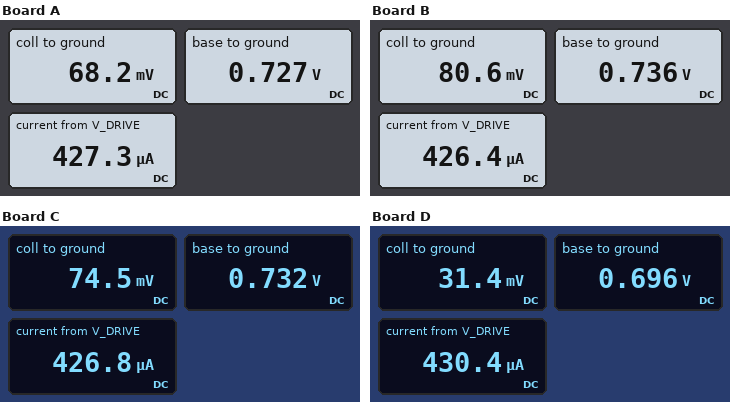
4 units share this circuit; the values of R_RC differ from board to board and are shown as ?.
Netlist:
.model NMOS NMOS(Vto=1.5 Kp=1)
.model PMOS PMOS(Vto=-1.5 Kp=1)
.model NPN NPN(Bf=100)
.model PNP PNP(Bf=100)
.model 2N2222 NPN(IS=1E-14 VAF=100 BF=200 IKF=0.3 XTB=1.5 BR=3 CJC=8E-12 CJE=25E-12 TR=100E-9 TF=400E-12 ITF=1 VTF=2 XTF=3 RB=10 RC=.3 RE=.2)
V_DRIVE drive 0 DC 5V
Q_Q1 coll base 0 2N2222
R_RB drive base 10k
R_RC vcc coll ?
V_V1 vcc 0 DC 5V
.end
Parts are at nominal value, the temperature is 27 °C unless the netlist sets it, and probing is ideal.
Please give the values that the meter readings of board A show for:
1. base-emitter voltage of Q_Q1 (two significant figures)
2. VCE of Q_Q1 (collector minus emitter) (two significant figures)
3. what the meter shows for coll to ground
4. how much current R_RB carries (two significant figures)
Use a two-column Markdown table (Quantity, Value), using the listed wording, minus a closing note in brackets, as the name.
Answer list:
| Quantity | Value |
|---|---|
| base-emitter voltage of Q_Q1 | 730 mV |
| VCE of Q_Q1 (collector minus emitter) | 68 mV |
| what the meter shows for coll to ground | 68.2 mV |
| how much current R_RB carries | 430 µA |
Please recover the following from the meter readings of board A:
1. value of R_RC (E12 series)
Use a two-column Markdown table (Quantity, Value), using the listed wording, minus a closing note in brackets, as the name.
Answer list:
| Quantity | Value |
|---|---|
| value of R_RC | 470 Ω |
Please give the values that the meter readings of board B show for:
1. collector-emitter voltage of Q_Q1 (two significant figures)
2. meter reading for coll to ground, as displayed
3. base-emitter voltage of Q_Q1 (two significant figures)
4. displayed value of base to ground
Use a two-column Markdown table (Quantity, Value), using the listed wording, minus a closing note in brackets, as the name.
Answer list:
| Quantity | Value |
|---|---|
| collector-emitter voltage of Q_Q1 | 81 mV |
| meter reading for coll to ground, as displayed | 80.6 mV |
| base-emitter voltage of Q_Q1 | 740 mV |
| displayed value of base to ground | 0.736 V |
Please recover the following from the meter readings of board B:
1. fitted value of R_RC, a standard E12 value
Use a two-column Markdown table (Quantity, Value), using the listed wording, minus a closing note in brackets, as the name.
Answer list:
| Quantity | Value |
|---|---|
| fitted value of R_RC, a standard E12 value | 330 Ω |
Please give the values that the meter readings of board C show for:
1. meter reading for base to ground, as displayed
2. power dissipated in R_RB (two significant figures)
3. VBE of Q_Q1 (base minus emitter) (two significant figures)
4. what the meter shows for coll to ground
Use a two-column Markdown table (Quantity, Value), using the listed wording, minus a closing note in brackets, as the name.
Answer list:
| Quantity | Value |
|---|---|
| meter reading for base to ground, as displayed | 0.732 V |
| power dissipated in R_RB | 1.8 mW |
| VBE of Q_Q1 (base minus emitter) | 730 mV |
| what the meter shows for coll to ground | 74.5 mV |
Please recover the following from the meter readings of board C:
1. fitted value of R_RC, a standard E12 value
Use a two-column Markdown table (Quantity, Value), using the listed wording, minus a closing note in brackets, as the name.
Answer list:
| Quantity | Value |
|---|---|
| fitted value of R_RC, a standard E12 value | 390 Ω |
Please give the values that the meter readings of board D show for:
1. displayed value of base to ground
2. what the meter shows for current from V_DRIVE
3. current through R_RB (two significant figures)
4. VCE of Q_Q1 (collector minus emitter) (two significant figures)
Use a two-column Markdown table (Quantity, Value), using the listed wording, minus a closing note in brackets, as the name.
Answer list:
| Quantity | Value |
|---|---|
| displayed value of base to ground | 0.696 V |
| what the meter shows for current from V_DRIVE | 430.4 µA |
| current through R_RB | 430 µA |
| VCE of Q_Q1 (collector minus emitter) | 31 mV |
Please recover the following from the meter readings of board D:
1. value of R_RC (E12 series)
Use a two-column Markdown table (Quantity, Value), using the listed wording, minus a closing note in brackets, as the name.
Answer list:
| Quantity | Value |
|---|---|
| value of R_RC | 2.2 kΩ |
